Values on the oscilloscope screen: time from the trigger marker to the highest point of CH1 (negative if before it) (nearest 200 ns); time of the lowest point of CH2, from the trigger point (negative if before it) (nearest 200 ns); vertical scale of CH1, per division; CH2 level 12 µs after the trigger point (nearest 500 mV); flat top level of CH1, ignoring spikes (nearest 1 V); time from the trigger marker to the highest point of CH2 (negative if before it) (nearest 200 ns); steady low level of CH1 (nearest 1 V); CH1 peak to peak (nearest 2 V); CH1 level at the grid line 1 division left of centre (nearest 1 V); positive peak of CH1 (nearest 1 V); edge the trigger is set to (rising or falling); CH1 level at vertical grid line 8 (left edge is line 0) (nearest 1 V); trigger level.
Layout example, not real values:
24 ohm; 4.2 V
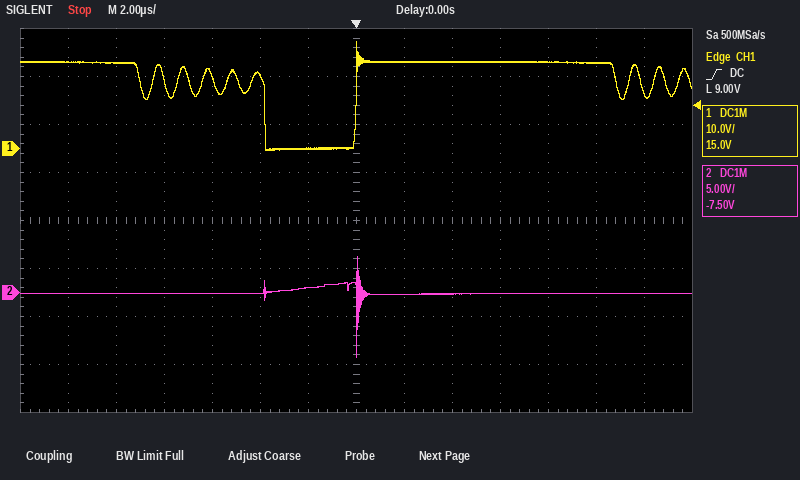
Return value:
0.0 µs; 0.0 µs; 10 V; 0.0 V; 18 V; 0.0 µs; 0 V; 22 V; 0 V; 22 V; rising; 18 V; 9.00 V
